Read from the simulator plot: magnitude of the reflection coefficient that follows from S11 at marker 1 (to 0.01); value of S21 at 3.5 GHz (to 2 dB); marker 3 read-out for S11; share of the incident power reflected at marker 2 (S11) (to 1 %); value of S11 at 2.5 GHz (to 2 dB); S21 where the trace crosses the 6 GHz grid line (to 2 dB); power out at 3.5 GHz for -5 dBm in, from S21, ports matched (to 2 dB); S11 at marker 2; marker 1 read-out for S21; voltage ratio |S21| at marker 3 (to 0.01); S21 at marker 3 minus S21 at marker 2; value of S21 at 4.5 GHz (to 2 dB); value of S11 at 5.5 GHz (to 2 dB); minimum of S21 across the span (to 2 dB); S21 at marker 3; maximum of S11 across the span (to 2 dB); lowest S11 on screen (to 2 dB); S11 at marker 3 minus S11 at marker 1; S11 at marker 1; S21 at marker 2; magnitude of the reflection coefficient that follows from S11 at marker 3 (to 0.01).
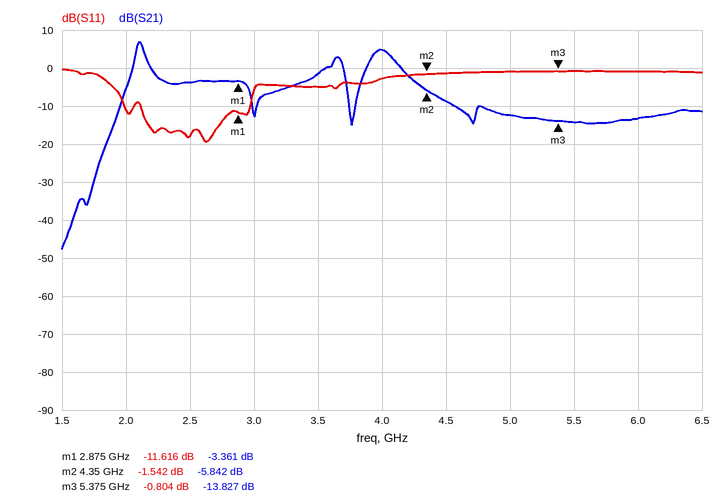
0.26
-2 dB
-0.804 dB
70 %
-18 dB
-14 dB
-6 dBm
-1.542 dB
-3.361 dB
0.20
-7.985 dB
-8 dB
0 dB
-48 dB
-13.827 dB
0 dB
-20 dB
10.812 dB
-11.616 dB
-5.842 dB
0.91
